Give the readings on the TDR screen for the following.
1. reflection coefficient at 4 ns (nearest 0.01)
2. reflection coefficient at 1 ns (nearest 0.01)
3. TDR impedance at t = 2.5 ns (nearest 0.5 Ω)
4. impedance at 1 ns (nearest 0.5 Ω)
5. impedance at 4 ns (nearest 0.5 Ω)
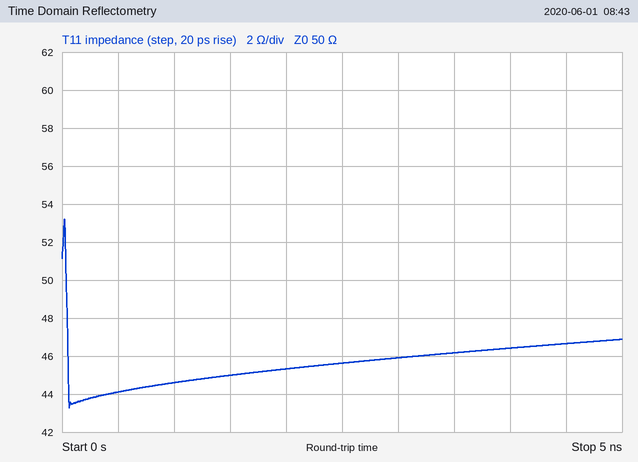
-0.04
-0.06
45.5 Ω
44.5 Ω
46.5 Ω
